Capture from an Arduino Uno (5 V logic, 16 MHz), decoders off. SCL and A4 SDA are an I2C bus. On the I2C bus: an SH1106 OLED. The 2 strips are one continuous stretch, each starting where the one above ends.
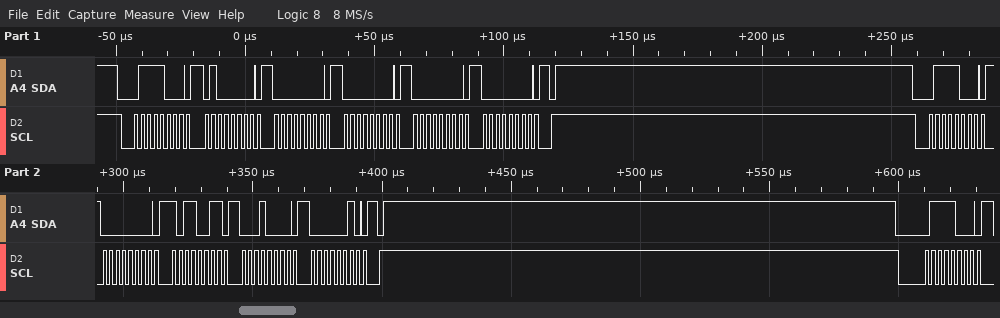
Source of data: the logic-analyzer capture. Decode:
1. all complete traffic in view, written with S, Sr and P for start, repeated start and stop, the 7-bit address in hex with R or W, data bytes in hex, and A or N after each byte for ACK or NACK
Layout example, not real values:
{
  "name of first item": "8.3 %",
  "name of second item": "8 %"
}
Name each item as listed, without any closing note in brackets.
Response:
{
  "all complete traffic in view, written with S, Sr and P for start, repeated start and stop, the 7-bit address in hex with R or W, data bytes in hex, and A or N after each byte for ACK or NACK": "S 3CW A 40 A 00 A 00 A 00 A 00 A P S 3CW A 00 A B3 A 10 A 02 A P S 3CW A"
}
